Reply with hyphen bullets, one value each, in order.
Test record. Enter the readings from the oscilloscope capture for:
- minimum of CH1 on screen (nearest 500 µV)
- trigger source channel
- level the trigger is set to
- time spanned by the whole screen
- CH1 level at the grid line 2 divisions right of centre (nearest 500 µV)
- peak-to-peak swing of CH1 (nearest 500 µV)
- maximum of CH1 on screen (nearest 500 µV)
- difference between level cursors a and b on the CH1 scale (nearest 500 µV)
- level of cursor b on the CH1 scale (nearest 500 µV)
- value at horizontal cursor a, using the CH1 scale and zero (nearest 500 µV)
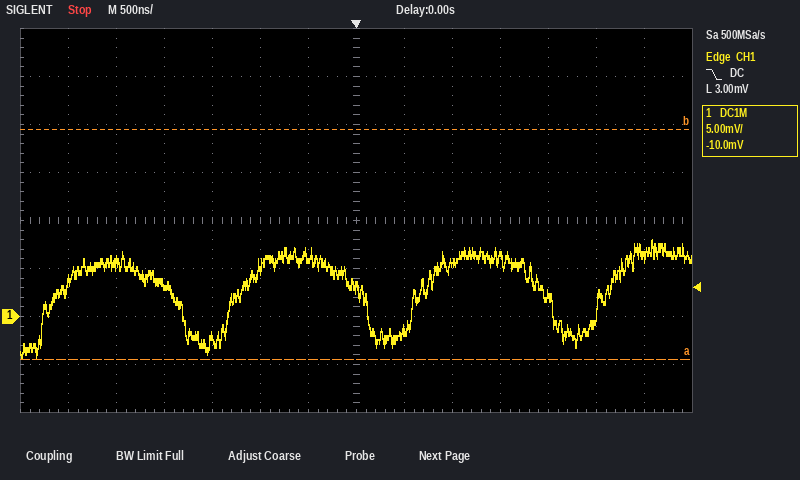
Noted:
- -4.5 mV
- CH1
- 3.00 mV
- 7 µs
- 5.5 mV
- 12.5 mV
- 8.0 mV
- 24.0 mV
- 19.5 mV
- -4.5 mV
